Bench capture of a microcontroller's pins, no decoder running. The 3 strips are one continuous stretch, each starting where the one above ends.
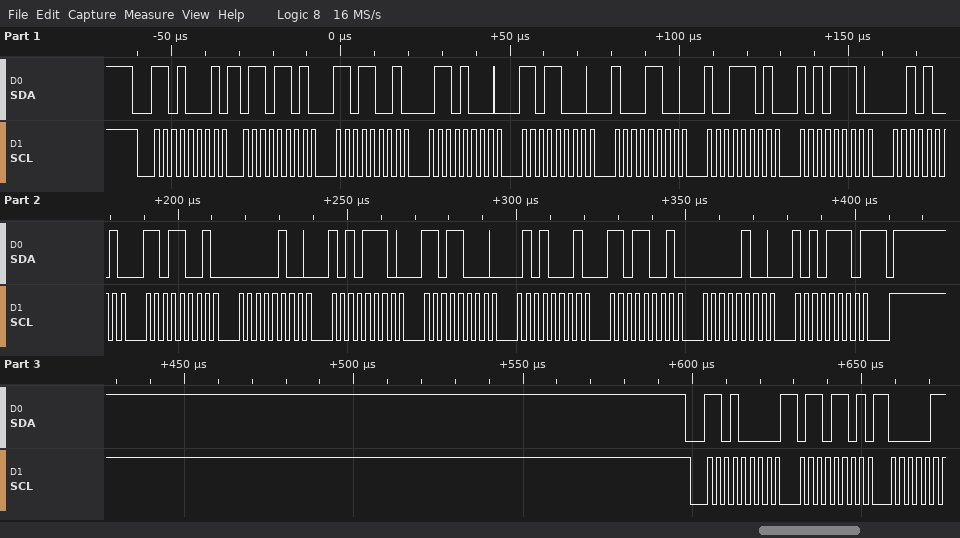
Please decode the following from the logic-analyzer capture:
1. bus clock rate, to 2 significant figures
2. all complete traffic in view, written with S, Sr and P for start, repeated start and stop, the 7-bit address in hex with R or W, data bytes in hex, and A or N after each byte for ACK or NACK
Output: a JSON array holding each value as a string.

["400 kHz", "S 68R A 6D A D9 A 68 A D8 A 8C A 9D A AE A 29 A D9 A 04 A AE A D8 A 51 A D9 A 04 A AE N P S 68W A 6D A"]
